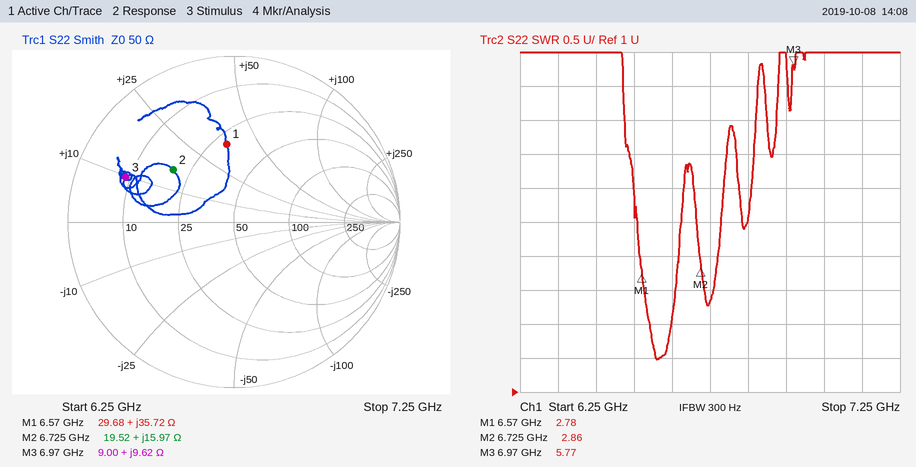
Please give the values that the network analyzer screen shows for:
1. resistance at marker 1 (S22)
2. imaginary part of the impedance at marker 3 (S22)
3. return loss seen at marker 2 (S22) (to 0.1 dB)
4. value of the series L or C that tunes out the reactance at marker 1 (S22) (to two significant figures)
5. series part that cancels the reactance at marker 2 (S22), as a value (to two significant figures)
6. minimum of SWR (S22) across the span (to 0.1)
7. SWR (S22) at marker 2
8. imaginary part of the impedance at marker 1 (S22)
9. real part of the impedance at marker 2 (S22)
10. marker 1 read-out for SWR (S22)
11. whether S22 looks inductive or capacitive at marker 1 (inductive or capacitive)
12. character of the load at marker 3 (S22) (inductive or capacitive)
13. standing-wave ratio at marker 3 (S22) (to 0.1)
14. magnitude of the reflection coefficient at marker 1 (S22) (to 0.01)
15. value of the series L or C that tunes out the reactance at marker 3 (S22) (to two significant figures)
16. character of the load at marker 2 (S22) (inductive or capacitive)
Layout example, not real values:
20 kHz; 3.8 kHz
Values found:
29.68 Ω; +9.62 Ω; 6.3 dB; 680 fF; 1.5 pF; 1.5; 2.86; +35.72 Ω; 19.52 Ω; 2.78; inductive; inductive; 5.8; 0.47; 2.4 pF; inductive
